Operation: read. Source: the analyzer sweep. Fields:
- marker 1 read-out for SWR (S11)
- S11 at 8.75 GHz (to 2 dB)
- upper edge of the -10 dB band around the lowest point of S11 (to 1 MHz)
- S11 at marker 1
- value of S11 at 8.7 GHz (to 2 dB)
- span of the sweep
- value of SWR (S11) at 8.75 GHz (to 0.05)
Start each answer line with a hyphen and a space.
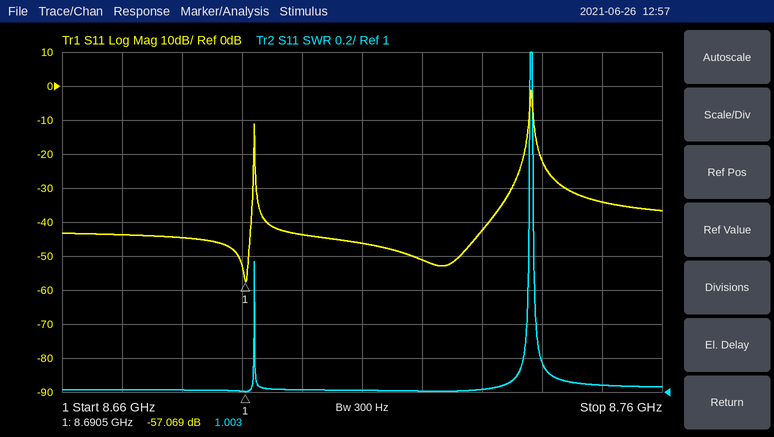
- 1.003
- -34 dB
- 8.738 GHz
- -57.069 dB
- -44 dB
- 100 MHz
- 1.05
